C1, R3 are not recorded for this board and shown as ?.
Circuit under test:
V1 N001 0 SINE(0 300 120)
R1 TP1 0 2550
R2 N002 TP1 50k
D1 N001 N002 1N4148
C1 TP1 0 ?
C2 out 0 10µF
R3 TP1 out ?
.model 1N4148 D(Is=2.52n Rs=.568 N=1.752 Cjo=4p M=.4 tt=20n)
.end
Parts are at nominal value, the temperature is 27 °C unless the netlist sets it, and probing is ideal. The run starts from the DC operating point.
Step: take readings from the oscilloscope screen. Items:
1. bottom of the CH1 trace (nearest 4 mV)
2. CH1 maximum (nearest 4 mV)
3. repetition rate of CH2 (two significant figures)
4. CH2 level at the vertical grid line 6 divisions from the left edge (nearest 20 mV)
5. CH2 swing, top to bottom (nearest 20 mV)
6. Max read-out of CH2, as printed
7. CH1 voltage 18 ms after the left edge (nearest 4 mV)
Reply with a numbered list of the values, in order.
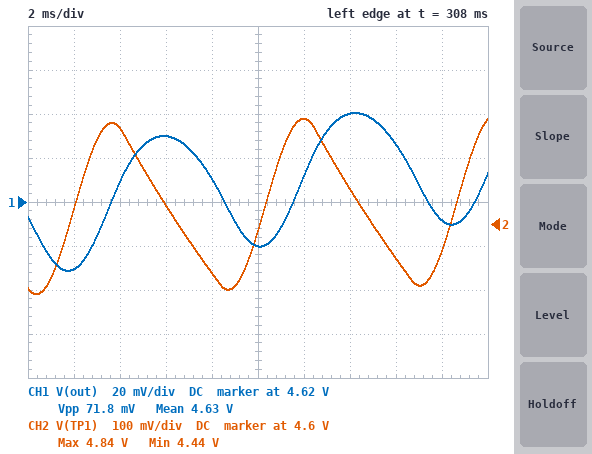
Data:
1. 4.588 V
2. 4.660 V
3. 120 Hz
4. 4.84 V
5. 400 mV
6. 4.84 V
7. 4.612 V
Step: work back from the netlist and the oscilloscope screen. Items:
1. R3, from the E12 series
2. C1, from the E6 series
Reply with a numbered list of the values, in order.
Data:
1. 820 Ω
2. 22 µF
